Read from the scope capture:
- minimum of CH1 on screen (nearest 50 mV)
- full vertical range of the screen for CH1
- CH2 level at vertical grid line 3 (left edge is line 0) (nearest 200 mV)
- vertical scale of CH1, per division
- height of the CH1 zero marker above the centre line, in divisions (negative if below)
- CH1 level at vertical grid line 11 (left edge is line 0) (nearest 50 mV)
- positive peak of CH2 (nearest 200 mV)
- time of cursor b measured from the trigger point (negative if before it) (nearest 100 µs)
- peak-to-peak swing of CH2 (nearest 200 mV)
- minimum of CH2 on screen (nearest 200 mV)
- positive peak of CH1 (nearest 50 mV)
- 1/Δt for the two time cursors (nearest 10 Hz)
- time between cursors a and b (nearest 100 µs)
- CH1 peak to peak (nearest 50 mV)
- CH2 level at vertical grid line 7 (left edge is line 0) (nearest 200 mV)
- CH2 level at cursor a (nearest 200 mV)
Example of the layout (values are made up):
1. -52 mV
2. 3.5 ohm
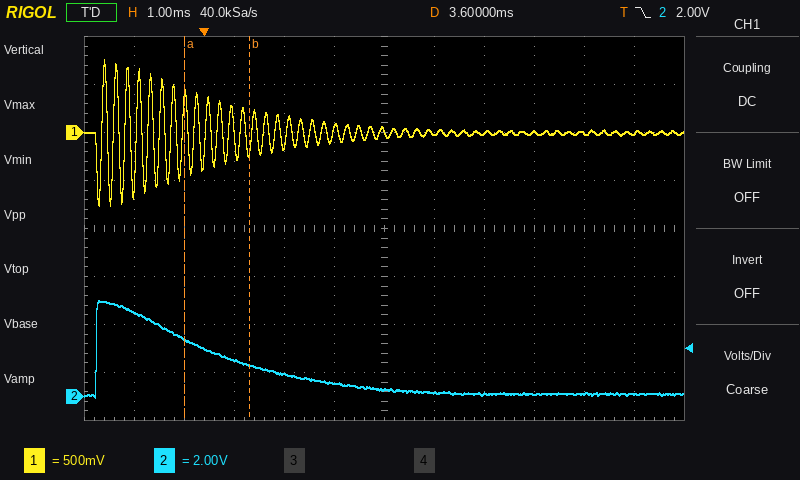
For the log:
1. -750 mV
2. 4 V
3. 1.6 V
4. 500 mV
5. +2.0 div
6. 0 mV
7. 4.0 V
8. +900 µs
9. 4.0 V
10. 0.0 V
11. 750 mV
12. 770 Hz
13. 1.3 ms
14. 1.50 V
15. 200 mV
16. 2.4 V
